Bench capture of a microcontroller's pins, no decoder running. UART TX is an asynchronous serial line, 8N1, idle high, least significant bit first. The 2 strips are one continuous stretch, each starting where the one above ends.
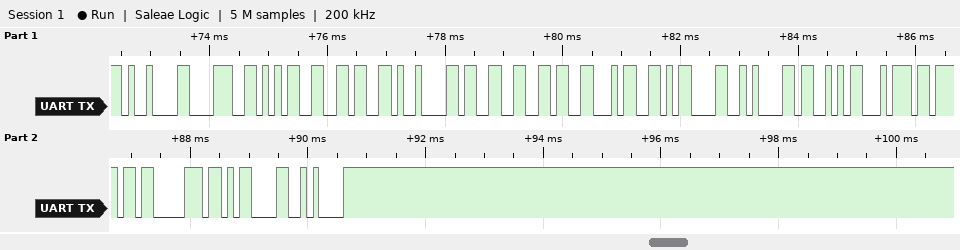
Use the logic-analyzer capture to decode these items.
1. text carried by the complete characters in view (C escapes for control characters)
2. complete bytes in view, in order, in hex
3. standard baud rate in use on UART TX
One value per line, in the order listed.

"\t856\t364\r\nStop\r\n"
09 38 35 36 09 33 36 34 0D 0A 53 74 6F 70 0D 0A
9600 baud
